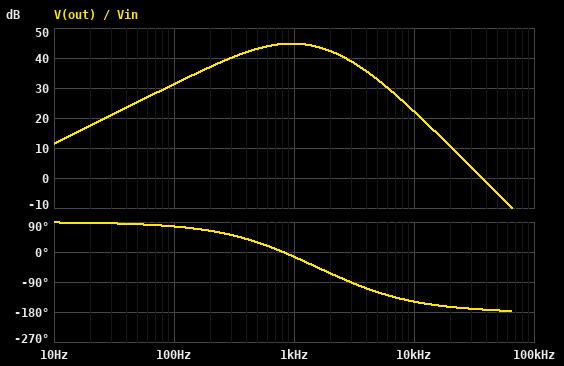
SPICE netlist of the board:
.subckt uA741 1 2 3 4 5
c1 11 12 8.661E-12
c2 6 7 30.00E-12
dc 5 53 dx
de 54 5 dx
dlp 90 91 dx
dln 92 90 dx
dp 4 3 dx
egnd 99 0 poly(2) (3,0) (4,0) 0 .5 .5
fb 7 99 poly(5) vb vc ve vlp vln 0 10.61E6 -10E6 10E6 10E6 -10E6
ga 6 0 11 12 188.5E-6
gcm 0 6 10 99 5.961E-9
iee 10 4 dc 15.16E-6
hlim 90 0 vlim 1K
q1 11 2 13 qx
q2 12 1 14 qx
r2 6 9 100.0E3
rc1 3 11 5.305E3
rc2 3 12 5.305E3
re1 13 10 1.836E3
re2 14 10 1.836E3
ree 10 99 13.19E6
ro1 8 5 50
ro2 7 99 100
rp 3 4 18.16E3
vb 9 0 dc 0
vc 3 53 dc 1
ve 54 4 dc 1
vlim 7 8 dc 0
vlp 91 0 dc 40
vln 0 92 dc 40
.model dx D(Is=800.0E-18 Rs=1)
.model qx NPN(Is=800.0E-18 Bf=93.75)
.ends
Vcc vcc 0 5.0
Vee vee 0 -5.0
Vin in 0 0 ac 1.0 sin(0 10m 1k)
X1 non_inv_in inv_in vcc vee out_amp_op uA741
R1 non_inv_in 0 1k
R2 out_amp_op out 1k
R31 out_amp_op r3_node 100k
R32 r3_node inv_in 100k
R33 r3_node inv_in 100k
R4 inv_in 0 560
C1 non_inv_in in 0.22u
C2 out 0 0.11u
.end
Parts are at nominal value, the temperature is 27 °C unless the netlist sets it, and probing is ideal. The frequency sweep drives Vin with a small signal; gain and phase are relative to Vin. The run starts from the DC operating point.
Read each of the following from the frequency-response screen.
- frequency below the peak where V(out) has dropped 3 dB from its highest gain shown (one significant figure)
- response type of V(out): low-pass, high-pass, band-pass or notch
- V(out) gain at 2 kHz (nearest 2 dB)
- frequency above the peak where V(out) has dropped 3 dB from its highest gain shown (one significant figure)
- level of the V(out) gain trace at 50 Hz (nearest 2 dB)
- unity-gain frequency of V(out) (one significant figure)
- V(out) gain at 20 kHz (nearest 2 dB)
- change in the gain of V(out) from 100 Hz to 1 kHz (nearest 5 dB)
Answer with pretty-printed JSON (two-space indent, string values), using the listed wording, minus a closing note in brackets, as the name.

{
  "frequency below the peak where V(out) has dropped 3 dB from its highest gain shown": "400 Hz",
  "response type of V(out): low-pass, high-pass, band-pass or notch": "band-pass",
  "V(out) gain at 2 kHz": "42 dB",
  "frequency above the peak where V(out) has dropped 3 dB from its highest gain shown": "2 kHz",
  "level of the V(out) gain trace at 50 Hz": "26 dB",
  "unity-gain frequency of V(out)": "40 kHz",
  "V(out) gain at 20 kHz": "10 dB",
  "change in the gain of V(out) from 100 Hz to 1 kHz": "15 dB"
}
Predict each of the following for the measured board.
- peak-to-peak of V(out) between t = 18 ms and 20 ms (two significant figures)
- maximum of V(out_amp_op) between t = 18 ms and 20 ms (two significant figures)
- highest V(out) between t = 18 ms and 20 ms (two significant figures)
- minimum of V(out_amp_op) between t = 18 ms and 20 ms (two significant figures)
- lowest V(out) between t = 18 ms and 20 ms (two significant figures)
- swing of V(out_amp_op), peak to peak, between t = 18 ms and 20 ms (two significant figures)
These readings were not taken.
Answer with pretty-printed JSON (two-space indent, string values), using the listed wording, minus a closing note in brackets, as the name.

{
  "peak-to-peak of V(out) between t = 18 ms and 20 ms": "3.5 V",
  "maximum of V(out_amp_op) between t = 18 ms and 20 ms": "2.1 V",
  "highest V(out) between t = 18 ms and 20 ms": "1.7 V",
  "minimum of V(out_amp_op) between t = 18 ms and 20 ms": "-2.1 V",
  "lowest V(out) between t = 18 ms and 20 ms": "-1.7 V",
  "swing of V(out_amp_op), peak to peak, between t = 18 ms and 20 ms": "4.2 V"
}
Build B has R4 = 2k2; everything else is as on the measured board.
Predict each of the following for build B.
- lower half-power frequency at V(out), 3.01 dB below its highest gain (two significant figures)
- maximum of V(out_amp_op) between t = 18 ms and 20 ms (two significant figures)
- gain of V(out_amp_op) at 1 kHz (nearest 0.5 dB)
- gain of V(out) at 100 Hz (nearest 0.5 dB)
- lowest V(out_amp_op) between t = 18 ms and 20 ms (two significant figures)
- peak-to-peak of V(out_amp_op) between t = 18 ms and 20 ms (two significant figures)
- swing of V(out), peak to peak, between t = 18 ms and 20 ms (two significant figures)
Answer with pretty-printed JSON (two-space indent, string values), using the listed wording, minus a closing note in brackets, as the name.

{
  "lower half-power frequency at V(out), 3.01 dB below its highest gain": "410 Hz",
  "maximum of V(out_amp_op) between t = 18 ms and 20 ms": "570 mV",
  "gain of V(out_amp_op) at 1 kHz": "35.0 dB",
  "gain of V(out) at 100 Hz": "19.5 dB",
  "lowest V(out_amp_op) between t = 18 ms and 20 ms": "-550 mV",
  "peak-to-peak of V(out_amp_op) between t = 18 ms and 20 ms": "1.1 V",
  "swing of V(out), peak to peak, between t = 18 ms and 20 ms": "920 mV"
}
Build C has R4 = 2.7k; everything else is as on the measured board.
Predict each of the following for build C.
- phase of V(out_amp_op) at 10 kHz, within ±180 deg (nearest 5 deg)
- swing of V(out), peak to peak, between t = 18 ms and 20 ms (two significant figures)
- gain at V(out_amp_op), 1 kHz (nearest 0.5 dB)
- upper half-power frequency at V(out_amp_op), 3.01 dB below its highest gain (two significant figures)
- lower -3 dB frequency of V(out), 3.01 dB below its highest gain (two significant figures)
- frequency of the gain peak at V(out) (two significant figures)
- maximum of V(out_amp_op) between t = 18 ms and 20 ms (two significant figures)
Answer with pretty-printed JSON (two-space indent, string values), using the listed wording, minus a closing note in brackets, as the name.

{
  "phase of V(out_amp_op) at 10 kHz, within ±180 deg": "-25 deg",
  "swing of V(out), peak to peak, between t = 18 ms and 20 ms": "750 mV",
  "gain at V(out_amp_op), 1 kHz": "33.0 dB",
  "upper half-power frequency at V(out_amp_op), 3.01 dB below its highest gain": "18 kHz",
  "lower -3 dB frequency of V(out), 3.01 dB below its highest gain": "410 Hz",
  "frequency of the gain peak at V(out)": "1.0 kHz",
  "maximum of V(out_amp_op) between t = 18 ms and 20 ms": "470 mV"
}
